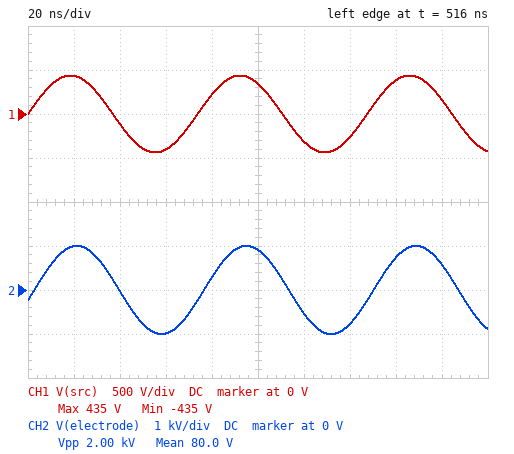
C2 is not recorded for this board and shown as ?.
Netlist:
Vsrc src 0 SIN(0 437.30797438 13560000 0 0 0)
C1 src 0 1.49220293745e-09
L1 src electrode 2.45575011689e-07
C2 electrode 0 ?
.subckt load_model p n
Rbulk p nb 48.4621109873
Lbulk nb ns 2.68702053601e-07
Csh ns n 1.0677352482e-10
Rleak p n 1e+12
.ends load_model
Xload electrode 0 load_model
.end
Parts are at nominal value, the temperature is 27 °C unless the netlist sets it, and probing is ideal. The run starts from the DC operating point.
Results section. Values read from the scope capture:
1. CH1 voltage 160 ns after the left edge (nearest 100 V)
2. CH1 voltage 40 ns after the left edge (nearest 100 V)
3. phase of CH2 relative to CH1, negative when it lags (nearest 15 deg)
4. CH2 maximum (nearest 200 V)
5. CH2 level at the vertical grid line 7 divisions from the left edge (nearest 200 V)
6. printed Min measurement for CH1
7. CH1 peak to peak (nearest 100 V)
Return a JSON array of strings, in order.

["400 V", "-100 V", "-15 deg", "1.0 kV", "-800 V", "-435 V", "900 V"]
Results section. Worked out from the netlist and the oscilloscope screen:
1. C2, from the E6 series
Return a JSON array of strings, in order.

["220 pF"]
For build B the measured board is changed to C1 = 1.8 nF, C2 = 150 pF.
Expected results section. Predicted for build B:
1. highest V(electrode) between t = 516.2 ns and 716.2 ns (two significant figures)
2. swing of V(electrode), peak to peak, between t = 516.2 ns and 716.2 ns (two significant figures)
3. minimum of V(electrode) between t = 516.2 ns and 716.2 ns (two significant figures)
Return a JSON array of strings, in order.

["780 V", "1.6 kV", "-780 V"]
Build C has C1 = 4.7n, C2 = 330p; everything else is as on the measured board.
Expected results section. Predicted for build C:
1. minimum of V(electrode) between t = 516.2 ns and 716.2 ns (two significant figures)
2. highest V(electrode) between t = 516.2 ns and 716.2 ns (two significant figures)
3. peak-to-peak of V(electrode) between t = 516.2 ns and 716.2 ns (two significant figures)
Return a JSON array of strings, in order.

["-1.7 kV", "1.7 kV", "3.5 kV"]
